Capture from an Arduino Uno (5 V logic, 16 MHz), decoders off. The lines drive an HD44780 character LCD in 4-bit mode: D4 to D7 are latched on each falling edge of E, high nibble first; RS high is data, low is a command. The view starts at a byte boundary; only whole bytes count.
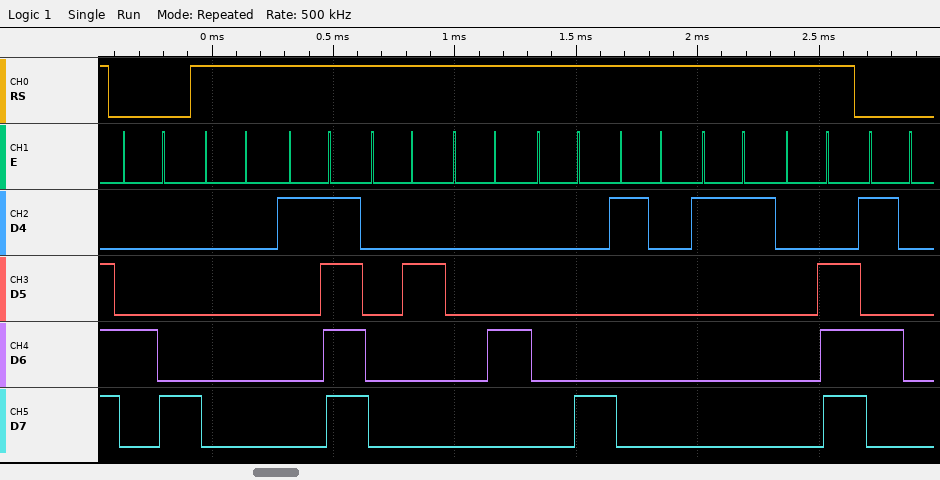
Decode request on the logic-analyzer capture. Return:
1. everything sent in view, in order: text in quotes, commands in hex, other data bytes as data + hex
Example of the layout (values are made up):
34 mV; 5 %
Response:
0x48 data 00 1F 02 04 08 10 11 0E 0x50
